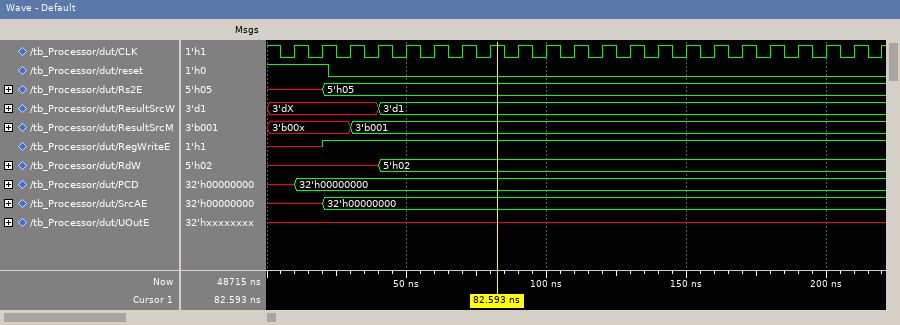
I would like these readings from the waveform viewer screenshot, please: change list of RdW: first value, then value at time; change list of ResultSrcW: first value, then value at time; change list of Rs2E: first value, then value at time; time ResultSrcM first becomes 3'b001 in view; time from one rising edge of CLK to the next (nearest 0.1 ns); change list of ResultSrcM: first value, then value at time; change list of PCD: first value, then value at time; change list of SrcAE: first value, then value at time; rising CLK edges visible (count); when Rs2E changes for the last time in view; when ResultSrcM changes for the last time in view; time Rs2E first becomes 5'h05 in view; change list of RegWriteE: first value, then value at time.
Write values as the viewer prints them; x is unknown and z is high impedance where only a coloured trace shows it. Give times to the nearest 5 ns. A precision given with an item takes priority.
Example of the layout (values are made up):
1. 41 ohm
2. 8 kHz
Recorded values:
1. x, 5'h02 at 40 ns
2. 3'dX, 3'd1 at 40 ns
3. x, 5'h05 at 20 ns
4. 30 ns
5. 10 ns
6. 3'b00x, 3'b001 at 30 ns
7. x, 32'h00000000 at 10 ns
8. x, 32'h00000000 at 20 ns
9. 22
10. 20 ns
11. 30 ns
12. 20 ns
13. x, 1 at 20 ns
